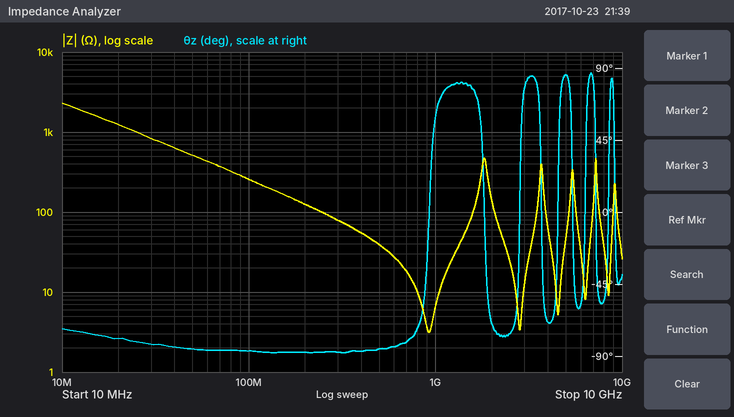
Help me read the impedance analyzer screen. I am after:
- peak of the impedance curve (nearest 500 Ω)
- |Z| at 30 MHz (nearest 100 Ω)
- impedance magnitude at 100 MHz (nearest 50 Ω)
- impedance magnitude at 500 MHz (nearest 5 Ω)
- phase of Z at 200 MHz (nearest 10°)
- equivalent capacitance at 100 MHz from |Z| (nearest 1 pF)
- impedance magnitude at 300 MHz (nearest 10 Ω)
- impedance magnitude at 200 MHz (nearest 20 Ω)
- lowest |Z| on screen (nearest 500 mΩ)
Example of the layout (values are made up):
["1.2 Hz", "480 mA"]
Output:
["2.5 kΩ", "800 Ω", "250 Ω", "40 Ω", "-90°", "6 pF", "80 Ω", "120 Ω", "3.0 Ω"]
